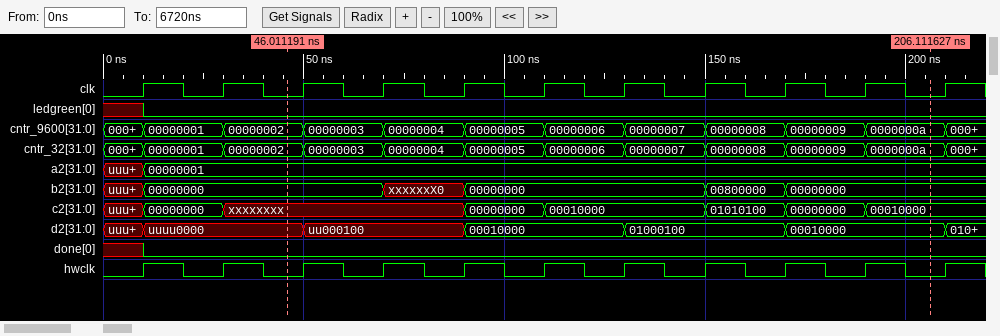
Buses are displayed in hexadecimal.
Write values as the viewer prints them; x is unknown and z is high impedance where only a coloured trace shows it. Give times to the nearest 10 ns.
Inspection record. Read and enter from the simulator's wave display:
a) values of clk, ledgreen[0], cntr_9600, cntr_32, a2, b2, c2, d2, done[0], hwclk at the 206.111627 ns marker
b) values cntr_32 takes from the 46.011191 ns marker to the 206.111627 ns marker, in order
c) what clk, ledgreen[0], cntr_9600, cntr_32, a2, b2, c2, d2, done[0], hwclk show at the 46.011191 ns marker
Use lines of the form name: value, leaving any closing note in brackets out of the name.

values of clk, ledgreen[0], cntr_9600, cntr_32, a2, b2, c2, d2, done[0], hwclk at the 206.111627 ns marker: clk=0, ledgreen[0]=0, cntr_9600=0000000a, cntr_32=0000000a, a2=00000001, b2=00000000, c2=00010000, d2=00010000, done[0]=0, hwclk=0
values cntr_32 takes from the 46.011191 ns marker to the 206.111627 ns marker, in order: 00000002, 00000003, 00000004, 00000005, 00000006, 00000007, 00000008, 00000009, 0000000a
what clk, ledgreen[0], cntr_9600, cntr_32, a2, b2, c2, d2, done[0], hwclk show at the 46.011191 ns marker: clk=0, ledgreen[0]=0, cntr_9600=00000002, cntr_32=00000002, a2=00000001, b2=00000000, c2=xxxxxxxx, d2=uuuu0000, done[0]=0, hwclk=0
